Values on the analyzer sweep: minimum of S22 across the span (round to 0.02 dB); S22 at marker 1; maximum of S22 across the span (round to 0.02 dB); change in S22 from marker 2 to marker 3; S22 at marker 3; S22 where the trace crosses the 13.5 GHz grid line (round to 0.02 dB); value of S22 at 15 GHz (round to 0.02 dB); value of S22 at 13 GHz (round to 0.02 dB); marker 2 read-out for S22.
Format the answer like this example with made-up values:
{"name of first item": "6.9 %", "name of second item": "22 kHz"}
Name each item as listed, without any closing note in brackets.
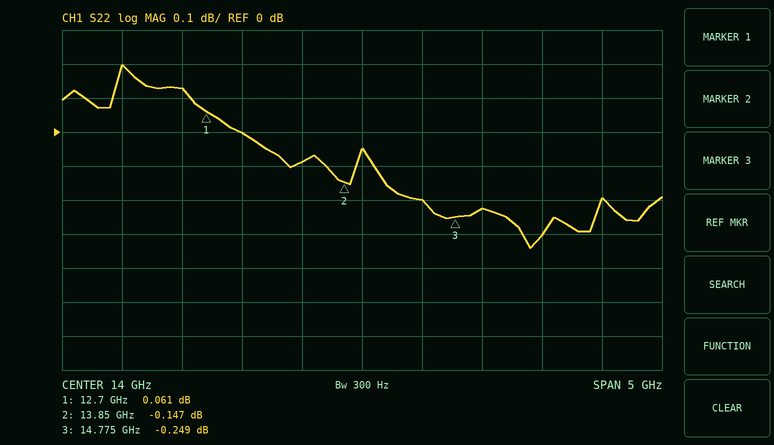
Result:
{"minimum of S22 across the span": "-0.34 dB", "S22 at marker 1": "0.061 dB", "maximum of S22 across the span": "0.20 dB", "change in S22 from marker 2 to marker 3": "-0.102 dB", "S22 at marker 3": "-0.249 dB", "S22 where the trace crosses the 13.5 GHz grid line": "-0.08 dB", "value of S22 at 15 GHz": "-0.22 dB", "value of S22 at 13 GHz": "0.00 dB", "marker 2 read-out for S22": "-0.147 dB"}
